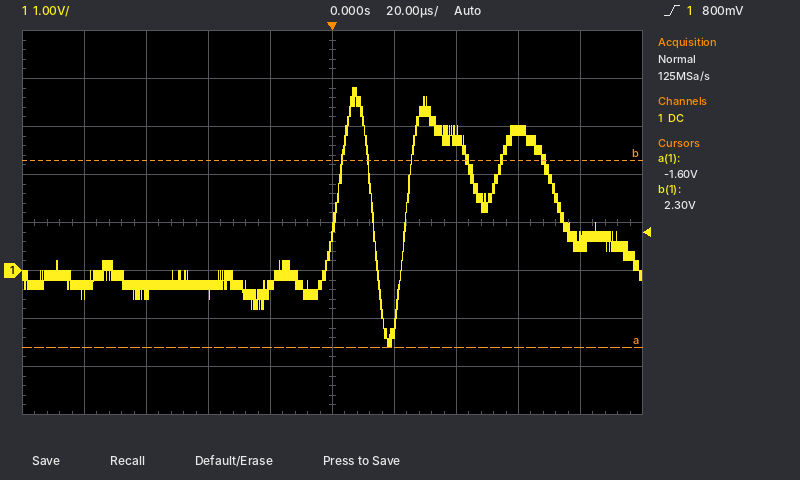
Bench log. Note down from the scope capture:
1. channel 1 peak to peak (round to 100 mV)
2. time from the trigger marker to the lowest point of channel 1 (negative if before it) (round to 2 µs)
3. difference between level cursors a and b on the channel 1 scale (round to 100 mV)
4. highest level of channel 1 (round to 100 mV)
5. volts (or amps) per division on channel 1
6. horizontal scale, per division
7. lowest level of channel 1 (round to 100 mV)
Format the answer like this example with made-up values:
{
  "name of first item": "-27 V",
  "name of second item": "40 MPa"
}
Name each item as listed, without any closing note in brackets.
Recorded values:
{
  "channel 1 peak to peak": "5.4 V",
  "time from the trigger marker to the lowest point of channel 1 (negative if before it)": "+18 µs",
  "difference between level cursors a and b on the channel 1 scale": "3.9 V",
  "highest level of channel 1": "3.8 V",
  "volts (or amps) per division on channel 1": "1 V",
  "horizontal scale, per division": "20 µs",
  "lowest level of channel 1": "-1.6 V"
}
